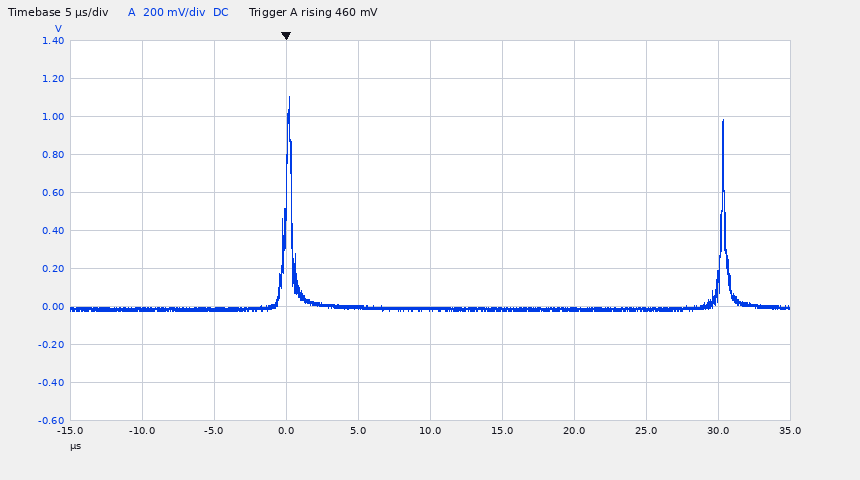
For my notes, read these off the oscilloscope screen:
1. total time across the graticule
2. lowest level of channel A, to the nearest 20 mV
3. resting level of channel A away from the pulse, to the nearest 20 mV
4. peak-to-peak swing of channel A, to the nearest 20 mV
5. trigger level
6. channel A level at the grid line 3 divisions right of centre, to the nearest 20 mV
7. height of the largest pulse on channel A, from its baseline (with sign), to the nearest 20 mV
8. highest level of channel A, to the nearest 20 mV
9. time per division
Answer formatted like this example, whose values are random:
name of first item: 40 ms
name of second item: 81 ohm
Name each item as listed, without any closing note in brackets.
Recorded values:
total time across the graticule: 50 µs
lowest level of channel A, to the nearest 20 mV: -20 mV
resting level of channel A away from the pulse, to the nearest 20 mV: -20 mV
peak-to-peak swing of channel A, to the nearest 20 mV: 1.12 V
trigger level: 460 mV
channel A level at the grid line 3 divisions right of centre, to the nearest 20 mV: -20 mV
height of the largest pulse on channel A, from its baseline (with sign), to the nearest 20 mV: +1.12 V
highest level of channel A, to the nearest 20 mV: 1.10 V
time per division: 5 µs
